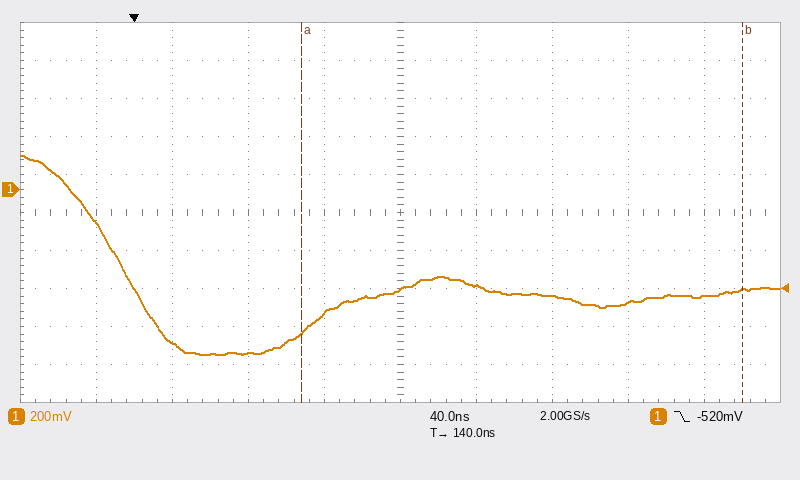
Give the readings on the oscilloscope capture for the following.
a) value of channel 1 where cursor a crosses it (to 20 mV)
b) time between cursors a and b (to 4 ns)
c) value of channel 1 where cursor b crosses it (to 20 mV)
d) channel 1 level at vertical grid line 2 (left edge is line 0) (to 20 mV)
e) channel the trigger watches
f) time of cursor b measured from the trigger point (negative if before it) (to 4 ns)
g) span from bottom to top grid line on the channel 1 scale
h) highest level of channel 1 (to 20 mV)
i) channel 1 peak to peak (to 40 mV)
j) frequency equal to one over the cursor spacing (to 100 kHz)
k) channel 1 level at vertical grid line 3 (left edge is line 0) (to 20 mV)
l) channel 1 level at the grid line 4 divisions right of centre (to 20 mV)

-760 mV
232 ns
-520 mV
-800 mV
channel 1
+320 ns
2 V
180 mV
1.04 V
4.3 MHz
-860 mV
-560 mV
